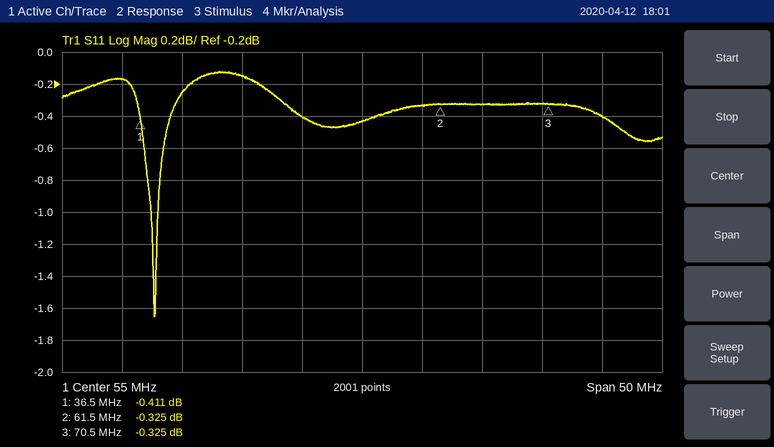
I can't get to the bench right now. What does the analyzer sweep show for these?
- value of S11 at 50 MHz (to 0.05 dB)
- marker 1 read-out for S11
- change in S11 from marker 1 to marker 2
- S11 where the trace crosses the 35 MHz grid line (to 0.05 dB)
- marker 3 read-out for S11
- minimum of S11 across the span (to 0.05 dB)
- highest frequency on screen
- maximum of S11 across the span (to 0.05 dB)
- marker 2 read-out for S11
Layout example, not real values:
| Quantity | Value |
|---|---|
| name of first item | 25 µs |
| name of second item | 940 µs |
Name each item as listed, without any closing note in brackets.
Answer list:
| Quantity | Value |
|---|---|
| value of S11 at 50 MHz | -0.40 dB |
| marker 1 read-out for S11 | -0.411 dB |
| change in S11 from marker 1 to marker 2 | 0.086 dB |
| S11 where the trace crosses the 35 MHz grid line | -0.15 dB |
| marker 3 read-out for S11 | -0.325 dB |
| minimum of S11 across the span | -1.65 dB |
| highest frequency on screen | 80 MHz |
| maximum of S11 across the span | -0.10 dB |
| marker 2 read-out for S11 | -0.325 dB |
